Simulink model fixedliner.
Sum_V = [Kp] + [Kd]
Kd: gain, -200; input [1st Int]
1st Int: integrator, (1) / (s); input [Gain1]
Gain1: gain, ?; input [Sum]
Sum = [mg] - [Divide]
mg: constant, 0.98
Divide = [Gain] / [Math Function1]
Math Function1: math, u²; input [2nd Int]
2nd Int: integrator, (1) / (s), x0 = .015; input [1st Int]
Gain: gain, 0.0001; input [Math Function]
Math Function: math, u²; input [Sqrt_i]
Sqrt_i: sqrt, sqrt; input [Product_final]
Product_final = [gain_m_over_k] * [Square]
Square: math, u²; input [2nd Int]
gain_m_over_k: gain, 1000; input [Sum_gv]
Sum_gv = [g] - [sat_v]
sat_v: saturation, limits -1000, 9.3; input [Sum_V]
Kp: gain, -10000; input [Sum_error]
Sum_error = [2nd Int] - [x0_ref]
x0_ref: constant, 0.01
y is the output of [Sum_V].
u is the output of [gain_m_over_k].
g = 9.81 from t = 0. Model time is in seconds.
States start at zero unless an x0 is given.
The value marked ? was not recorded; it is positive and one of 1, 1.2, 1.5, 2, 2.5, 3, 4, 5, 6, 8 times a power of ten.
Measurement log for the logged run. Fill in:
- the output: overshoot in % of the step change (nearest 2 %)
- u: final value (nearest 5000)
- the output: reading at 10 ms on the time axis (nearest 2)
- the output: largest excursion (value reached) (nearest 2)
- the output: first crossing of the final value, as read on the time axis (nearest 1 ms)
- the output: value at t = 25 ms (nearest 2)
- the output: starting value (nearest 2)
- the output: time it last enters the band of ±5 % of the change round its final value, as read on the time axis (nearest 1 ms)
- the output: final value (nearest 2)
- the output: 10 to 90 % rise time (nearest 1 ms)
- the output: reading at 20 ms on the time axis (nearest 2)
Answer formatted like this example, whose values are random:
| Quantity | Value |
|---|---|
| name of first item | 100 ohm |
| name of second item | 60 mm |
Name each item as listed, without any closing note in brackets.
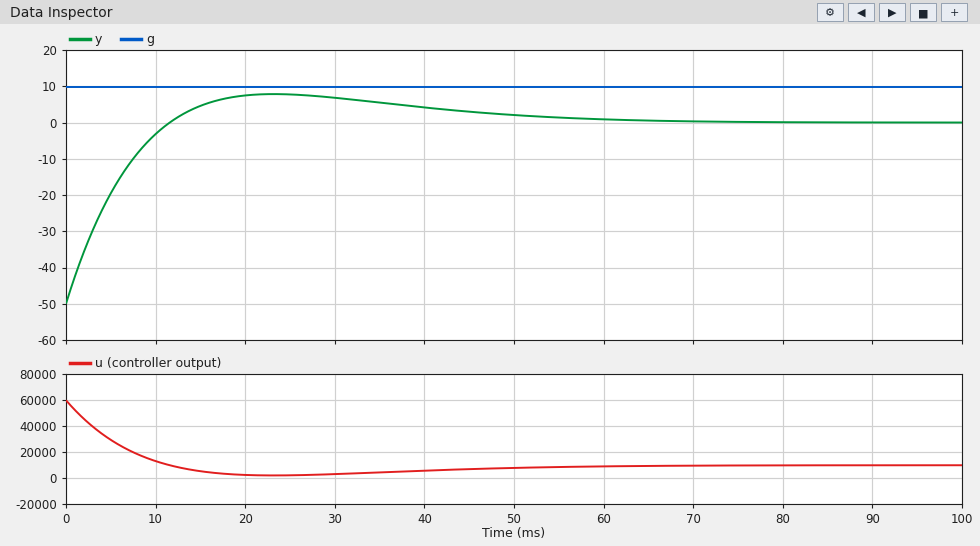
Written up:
| Quantity | Value |
|---|---|
| the output: overshoot in % of the step change | 16 % |
| u: final value | 10000 |
| the output: reading at 10 ms on the time axis | -4 |
| the output: largest excursion (value reached) | 8 |
| the output: first crossing of the final value, as read on the time axis | 12 ms |
| the output: value at t = 25 ms | 8 |
| the output: starting value | -50 |
| the output: time it last enters the band of ±5 % of the change round its final value, as read on the time axis | 47 ms |
| the output: final value | 0 |
| the output: 10 to 90 % rise time | 9 ms |
| the output: reading at 20 ms on the time axis | 8 |
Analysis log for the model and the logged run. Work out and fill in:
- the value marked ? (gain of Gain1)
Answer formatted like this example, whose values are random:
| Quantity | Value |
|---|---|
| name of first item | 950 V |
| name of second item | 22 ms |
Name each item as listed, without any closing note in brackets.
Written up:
| Quantity | Value |
|---|---|
| the value marked ? | 8 |
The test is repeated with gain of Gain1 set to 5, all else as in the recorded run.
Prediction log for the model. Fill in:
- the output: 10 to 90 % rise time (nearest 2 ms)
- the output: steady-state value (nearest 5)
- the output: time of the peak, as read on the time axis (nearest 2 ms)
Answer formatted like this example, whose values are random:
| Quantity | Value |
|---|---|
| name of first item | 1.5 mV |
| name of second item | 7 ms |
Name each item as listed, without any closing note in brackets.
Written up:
| Quantity | Value |
|---|---|
| the output: 10 to 90 % rise time | 12 ms |
| the output: steady-state value | 0 |
| the output: time of the peak, as read on the time axis | 34 ms |
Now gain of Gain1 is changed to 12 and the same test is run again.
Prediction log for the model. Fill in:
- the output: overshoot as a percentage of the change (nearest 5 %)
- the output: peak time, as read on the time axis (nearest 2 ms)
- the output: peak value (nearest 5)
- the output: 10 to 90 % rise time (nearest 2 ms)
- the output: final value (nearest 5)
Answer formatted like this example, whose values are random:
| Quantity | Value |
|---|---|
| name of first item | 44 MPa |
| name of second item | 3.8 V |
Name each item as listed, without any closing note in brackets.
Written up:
| Quantity | Value |
|---|---|
| the output: overshoot as a percentage of the change | 10 % |
| the output: peak time, as read on the time axis | 18 ms |
| the output: peak value | 5 |
| the output: 10 to 90 % rise time | 6 ms |
| the output: final value | 0 |
